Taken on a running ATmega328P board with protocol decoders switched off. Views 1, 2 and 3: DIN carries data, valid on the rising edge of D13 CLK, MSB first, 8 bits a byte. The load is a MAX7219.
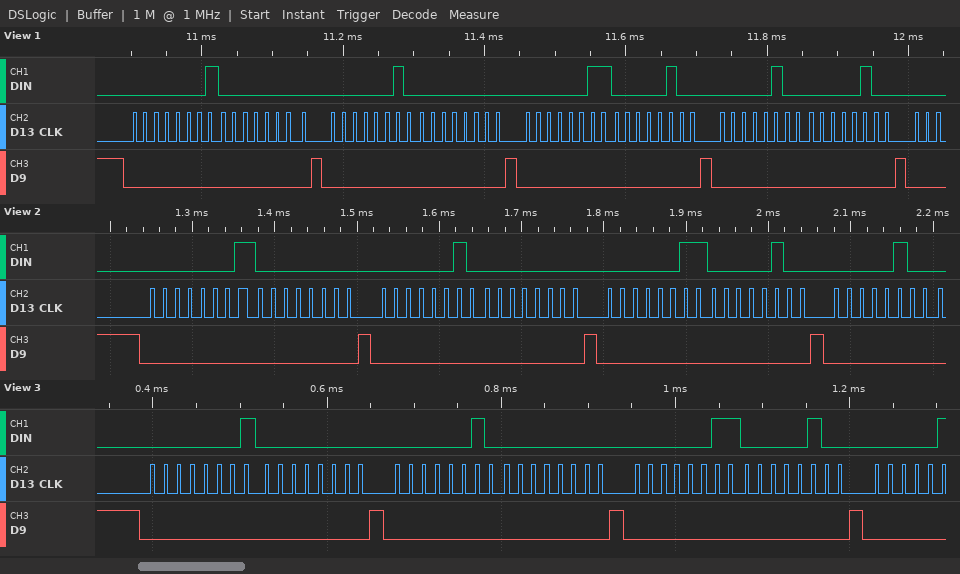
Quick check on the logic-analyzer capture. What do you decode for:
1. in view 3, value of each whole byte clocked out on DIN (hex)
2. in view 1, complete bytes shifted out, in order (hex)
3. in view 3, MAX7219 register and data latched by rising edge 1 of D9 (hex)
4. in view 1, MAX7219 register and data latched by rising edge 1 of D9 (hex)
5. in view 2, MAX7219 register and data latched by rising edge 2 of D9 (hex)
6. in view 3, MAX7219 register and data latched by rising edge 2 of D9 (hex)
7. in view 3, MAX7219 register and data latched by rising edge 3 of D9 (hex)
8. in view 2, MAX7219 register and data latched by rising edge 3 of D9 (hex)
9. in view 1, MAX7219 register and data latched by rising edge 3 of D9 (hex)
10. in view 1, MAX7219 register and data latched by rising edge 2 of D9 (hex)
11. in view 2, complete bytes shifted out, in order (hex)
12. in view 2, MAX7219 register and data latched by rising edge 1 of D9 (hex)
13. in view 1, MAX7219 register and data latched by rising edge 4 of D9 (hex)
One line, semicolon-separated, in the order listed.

01 00 02 00 03 04; 0x01 0x00 0x02 0x00 0x03 0x04 0x04 0x04; register 0x1, data 0x00; register 0x1, data 0x00; register 0x2, data 0x00; register 0x2, data 0x00; register 0x3, data 0x04; register 0x3, data 0x04; register 0x3, data 0x04; register 0x2, data 0x00; 01 00 02 00 03 04 04; register 0x1, data 0x00; register 0x4, data 0x04
